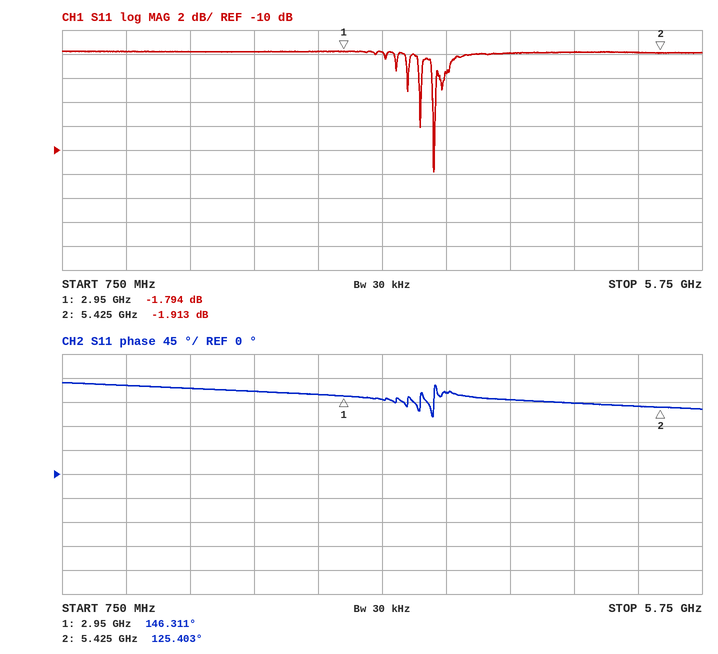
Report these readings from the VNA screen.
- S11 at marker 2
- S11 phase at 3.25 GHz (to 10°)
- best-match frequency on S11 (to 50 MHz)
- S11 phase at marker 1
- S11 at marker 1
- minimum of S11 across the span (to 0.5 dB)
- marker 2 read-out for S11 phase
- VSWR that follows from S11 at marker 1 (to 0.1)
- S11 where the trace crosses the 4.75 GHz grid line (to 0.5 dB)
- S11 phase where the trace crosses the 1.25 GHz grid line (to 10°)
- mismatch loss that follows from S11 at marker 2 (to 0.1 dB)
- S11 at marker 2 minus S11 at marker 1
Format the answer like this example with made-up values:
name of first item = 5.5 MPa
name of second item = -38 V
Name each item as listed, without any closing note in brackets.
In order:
S11 at marker 2 = -1.913 dB
S11 phase at 3.25 GHz = 140°
best-match frequency on S11 = 3.65 GHz
S11 phase at marker 1 = 146.311°
S11 at marker 1 = -1.794 dB
minimum of S11 across the span = -12.0 dB
marker 2 read-out for S11 phase = 125.403°
VSWR that follows from S11 at marker 1 = 9.7
S11 where the trace crosses the 4.75 GHz grid line = -2.0 dB
S11 phase where the trace crosses the 1.25 GHz grid line = 170°
mismatch loss that follows from S11 at marker 2 = 4.5 dB
S11 at marker 2 minus S11 at marker 1 = -0.119 dB
